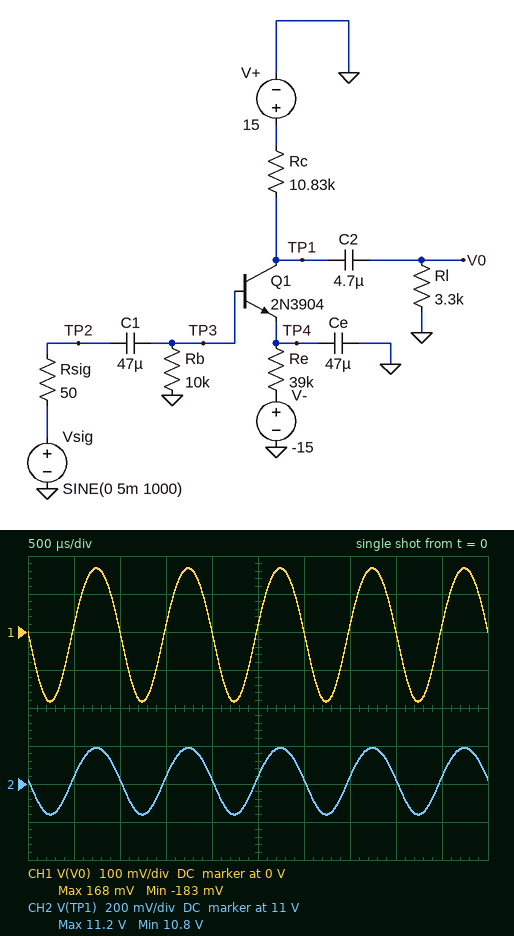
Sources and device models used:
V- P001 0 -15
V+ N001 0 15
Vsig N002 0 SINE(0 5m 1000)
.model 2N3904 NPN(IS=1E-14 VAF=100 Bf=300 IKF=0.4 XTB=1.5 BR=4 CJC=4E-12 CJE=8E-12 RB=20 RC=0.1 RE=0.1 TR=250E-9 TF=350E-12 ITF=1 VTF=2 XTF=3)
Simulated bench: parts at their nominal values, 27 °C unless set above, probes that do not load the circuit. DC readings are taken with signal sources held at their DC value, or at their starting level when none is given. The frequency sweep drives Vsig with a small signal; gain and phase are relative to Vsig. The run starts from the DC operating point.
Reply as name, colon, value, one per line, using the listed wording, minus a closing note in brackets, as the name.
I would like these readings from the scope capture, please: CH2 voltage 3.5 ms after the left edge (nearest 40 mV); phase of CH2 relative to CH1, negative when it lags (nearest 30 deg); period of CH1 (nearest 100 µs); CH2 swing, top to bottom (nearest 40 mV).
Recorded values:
CH2 voltage 3.5 ms after the left edge: 11.04 V
phase of CH2 relative to CH1, negative when it lags: 0 deg
period of CH1: 1.0 ms
CH2 swing, top to bottom: 360 mV
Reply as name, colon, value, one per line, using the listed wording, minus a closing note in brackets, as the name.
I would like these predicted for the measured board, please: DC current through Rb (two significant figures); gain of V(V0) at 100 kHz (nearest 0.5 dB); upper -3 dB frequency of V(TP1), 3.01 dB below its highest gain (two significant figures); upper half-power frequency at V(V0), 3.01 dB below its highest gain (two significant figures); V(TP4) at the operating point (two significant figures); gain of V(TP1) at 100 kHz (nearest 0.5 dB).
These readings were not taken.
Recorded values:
DC current through Rb: 1.1 µA
gain of V(V0) at 100 kHz: 31.0 dB
upper -3 dB frequency of V(TP1), 3.01 dB below its highest gain: 18 MHz
upper half-power frequency at V(V0), 3.01 dB below its highest gain: 18 MHz
V(TP4) at the operating point: -640 mV
gain of V(TP1) at 100 kHz: 31.0 dB
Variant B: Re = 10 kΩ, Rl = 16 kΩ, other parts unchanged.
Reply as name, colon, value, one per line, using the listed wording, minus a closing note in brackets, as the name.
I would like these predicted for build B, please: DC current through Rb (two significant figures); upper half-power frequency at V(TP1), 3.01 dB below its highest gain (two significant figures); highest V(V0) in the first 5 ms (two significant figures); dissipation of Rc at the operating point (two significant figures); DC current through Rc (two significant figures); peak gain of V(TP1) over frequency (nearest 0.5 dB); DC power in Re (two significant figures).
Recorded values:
DC current through Rb: 4.8 µA
upper half-power frequency at V(TP1), 3.01 dB below its highest gain: 1.1 MHz
highest V(V0) in the first 5 ms: 1.4 V
dissipation of Rc at the operating point: 22 mW
DC current through Rc: 1.4 mA
peak gain of V(TP1) over frequency: 50.0 dB
DC power in Re: 20 mW
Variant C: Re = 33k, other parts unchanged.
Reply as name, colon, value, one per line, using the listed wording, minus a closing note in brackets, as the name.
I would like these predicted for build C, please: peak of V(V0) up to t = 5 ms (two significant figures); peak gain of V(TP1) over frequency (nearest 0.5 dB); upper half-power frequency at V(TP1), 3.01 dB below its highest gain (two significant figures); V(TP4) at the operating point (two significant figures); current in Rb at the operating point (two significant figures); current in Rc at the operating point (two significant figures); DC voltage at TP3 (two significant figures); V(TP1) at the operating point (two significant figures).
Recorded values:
peak of V(V0) up to t = 5 ms: 200 mV
peak gain of V(TP1) over frequency: 32.5 dB
upper half-power frequency at V(TP1), 3.01 dB below its highest gain: 16 MHz
V(TP4) at the operating point: -640 mV
current in Rb at the operating point: 1.3 µA
current in Rc at the operating point: 430 µA
DC voltage at TP3: -13 mV
V(TP1) at the operating point: 10 V
